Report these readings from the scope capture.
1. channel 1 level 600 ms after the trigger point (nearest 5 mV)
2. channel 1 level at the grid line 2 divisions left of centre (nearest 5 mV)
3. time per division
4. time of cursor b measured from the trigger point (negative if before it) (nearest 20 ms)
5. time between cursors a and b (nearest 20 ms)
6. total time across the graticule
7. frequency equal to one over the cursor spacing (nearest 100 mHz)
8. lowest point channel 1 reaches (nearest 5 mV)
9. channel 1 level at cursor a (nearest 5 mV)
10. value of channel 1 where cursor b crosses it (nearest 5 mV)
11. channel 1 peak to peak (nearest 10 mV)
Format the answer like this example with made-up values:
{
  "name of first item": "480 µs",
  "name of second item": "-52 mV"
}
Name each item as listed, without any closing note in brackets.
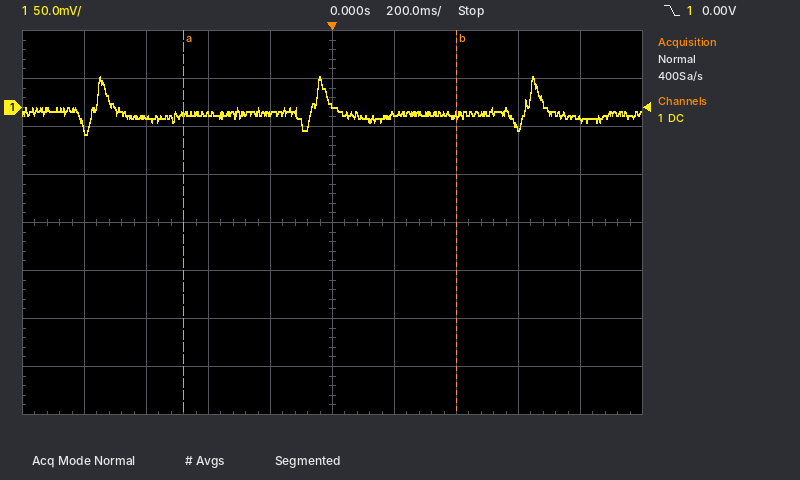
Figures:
{
  "channel 1 level 600 ms after the trigger point": "-20 mV",
  "channel 1 level at the grid line 2 divisions left of centre": "-5 mV",
  "time per division": "200 ms",
  "time of cursor b measured from the trigger point (negative if before it)": "+400 ms",
  "time between cursors a and b": "880 ms",
  "total time across the graticule": "2 s",
  "frequency equal to one over the cursor spacing": "1.1 Hz",
  "lowest point channel 1 reaches": "-30 mV",
  "channel 1 level at cursor a": "-5 mV",
  "value of channel 1 where cursor b crosses it": "-10 mV",
  "channel 1 peak to peak": "60 mV"
}
